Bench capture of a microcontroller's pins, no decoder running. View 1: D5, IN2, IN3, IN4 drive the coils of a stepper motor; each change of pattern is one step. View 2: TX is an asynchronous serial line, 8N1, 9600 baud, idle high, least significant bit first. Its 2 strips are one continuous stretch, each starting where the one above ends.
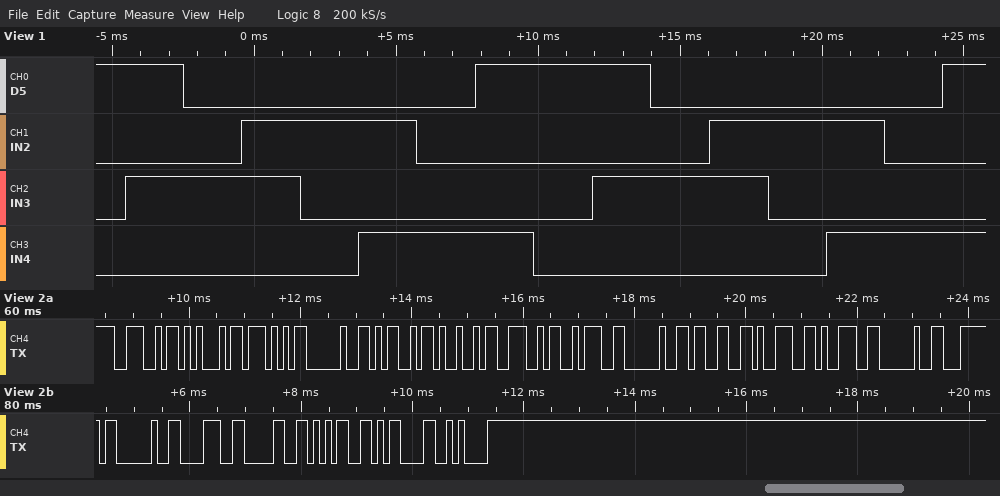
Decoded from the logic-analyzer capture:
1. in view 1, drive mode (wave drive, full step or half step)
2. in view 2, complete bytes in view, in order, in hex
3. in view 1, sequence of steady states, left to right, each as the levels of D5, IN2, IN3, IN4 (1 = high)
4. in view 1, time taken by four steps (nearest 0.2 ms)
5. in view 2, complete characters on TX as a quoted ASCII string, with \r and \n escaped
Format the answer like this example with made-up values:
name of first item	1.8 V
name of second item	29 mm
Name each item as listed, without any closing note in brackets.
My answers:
in view 1, drive mode	half step
in view 2, complete bytes in view, in order, in hex	4E 45 57 20 4D 49 4E 3A 20 33 39 39 20 7C 20 38 30 35 0D 0A
in view 1, sequence of steady states, left to right, each as the levels of D5, IN2, IN3, IN4	1000 1010 0010 0110 0100 0101 0001 1001 1000 1010 0010 0110 0100 0101 0001 1001
in view 1, time taken by four steps	8.2 ms
in view 2, complete characters on TX as a quoted ASCII string, with \r and \n escaped	"NEW MIN: 399 | 805\r\n"
